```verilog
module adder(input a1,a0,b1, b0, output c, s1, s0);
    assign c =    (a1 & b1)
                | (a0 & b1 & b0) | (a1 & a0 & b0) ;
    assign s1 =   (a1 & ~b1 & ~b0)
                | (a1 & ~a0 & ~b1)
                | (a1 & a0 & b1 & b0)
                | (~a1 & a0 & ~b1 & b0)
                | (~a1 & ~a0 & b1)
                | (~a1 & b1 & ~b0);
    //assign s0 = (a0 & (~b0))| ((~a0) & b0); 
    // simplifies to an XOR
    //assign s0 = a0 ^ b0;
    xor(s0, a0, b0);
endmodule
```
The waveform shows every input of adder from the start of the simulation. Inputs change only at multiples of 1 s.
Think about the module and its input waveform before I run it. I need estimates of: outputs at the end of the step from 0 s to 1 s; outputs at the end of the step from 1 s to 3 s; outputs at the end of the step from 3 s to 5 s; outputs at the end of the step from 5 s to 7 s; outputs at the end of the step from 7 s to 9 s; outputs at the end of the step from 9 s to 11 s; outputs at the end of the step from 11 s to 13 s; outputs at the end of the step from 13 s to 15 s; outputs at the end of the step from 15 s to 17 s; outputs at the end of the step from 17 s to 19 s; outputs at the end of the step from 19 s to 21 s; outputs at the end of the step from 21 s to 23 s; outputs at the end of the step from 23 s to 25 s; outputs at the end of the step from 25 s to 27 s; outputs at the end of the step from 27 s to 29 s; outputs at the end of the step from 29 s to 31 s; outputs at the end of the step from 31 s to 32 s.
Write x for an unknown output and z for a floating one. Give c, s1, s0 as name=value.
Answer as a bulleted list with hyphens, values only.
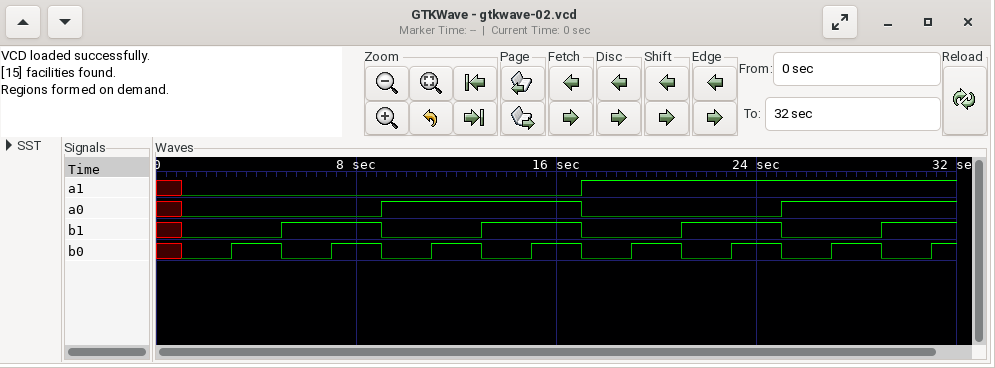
- c=x, s1=x, s0=x
- c=0, s1=0, s0=0
- c=0, s1=0, s0=1
- c=0, s1=1, s0=0
- c=0, s1=1, s0=1
- c=0, s1=0, s0=1
- c=0, s1=1, s0=0
- c=0, s1=1, s0=1
- c=1, s1=0, s0=0
- c=0, s1=1, s0=0
- c=0, s1=1, s0=1
- c=1, s1=0, s0=0
- c=1, s1=0, s0=1
- c=0, s1=1, s0=1
- c=1, s1=0, s0=0
- c=1, s1=0, s0=1
- c=1, s1=1, s0=0
